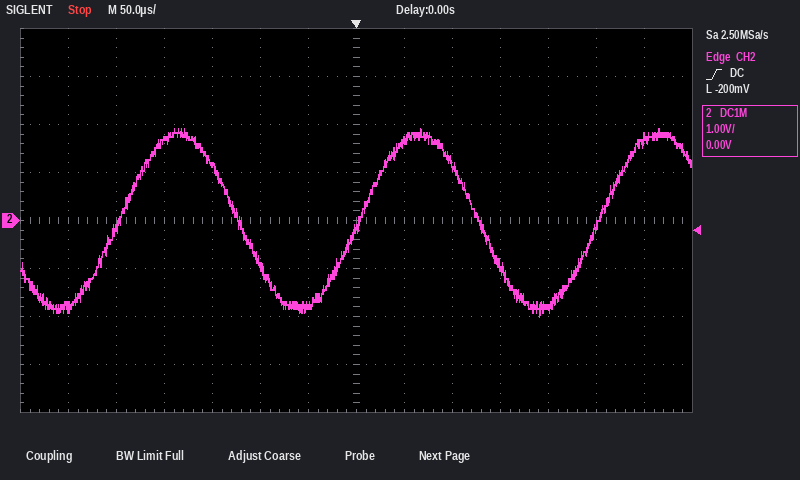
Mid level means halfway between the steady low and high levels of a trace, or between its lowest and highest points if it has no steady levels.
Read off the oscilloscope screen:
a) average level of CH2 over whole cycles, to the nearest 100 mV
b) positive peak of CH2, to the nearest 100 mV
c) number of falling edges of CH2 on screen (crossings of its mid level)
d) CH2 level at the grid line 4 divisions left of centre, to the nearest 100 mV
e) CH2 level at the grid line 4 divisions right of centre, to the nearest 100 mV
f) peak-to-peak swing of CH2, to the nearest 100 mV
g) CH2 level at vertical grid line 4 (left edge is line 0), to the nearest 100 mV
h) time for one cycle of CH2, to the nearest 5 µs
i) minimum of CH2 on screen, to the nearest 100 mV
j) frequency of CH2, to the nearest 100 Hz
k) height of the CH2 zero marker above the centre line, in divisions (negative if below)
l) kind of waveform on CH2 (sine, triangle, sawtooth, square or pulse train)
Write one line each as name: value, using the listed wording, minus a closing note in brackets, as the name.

average level of CH2 over whole cycles, to the nearest 100 mV: 0.0 V
positive peak of CH2, to the nearest 100 mV: 1.9 V
number of falling edges of CH2 on screen: 2
CH2 level at the grid line 4 divisions left of centre, to the nearest 100 mV: 1.7 V
CH2 level at the grid line 4 divisions right of centre, to the nearest 100 mV: -1.8 V
peak-to-peak swing of CH2, to the nearest 100 mV: 3.9 V
CH2 level at vertical grid line 4 (left edge is line 0), to the nearest 100 mV: 1.2 V
time for one cycle of CH2, to the nearest 5 µs: 250 µs
minimum of CH2 on screen, to the nearest 100 mV: -2.0 V
frequency of CH2, to the nearest 100 Hz: 4.0 kHz
height of the CH2 zero marker above the centre line, in divisions: 0.0 div
kind of waveform on CH2: sine
